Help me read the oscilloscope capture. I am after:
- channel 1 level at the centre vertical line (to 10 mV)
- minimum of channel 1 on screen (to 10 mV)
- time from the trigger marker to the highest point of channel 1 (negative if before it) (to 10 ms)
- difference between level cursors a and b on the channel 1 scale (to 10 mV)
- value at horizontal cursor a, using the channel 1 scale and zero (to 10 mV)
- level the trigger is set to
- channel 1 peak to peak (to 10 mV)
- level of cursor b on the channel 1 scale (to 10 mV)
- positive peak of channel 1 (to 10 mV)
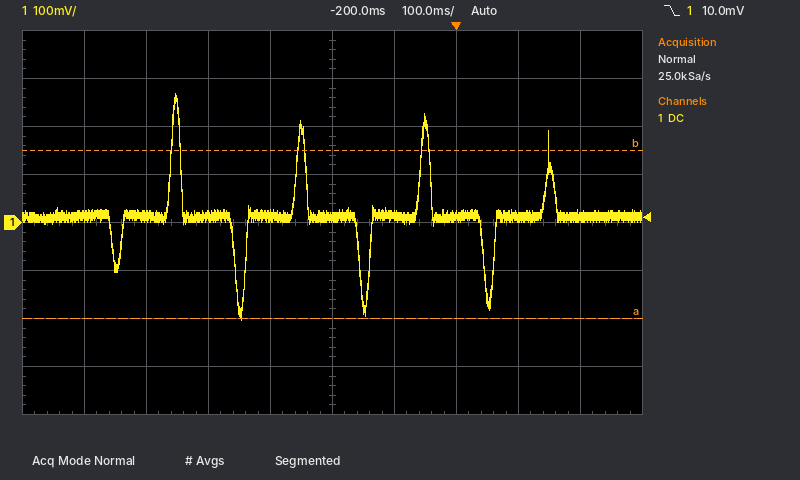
10 mV
-200 mV
-450 ms
350 mV
-200 mV
10.0 mV
470 mV
150 mV
270 mV
